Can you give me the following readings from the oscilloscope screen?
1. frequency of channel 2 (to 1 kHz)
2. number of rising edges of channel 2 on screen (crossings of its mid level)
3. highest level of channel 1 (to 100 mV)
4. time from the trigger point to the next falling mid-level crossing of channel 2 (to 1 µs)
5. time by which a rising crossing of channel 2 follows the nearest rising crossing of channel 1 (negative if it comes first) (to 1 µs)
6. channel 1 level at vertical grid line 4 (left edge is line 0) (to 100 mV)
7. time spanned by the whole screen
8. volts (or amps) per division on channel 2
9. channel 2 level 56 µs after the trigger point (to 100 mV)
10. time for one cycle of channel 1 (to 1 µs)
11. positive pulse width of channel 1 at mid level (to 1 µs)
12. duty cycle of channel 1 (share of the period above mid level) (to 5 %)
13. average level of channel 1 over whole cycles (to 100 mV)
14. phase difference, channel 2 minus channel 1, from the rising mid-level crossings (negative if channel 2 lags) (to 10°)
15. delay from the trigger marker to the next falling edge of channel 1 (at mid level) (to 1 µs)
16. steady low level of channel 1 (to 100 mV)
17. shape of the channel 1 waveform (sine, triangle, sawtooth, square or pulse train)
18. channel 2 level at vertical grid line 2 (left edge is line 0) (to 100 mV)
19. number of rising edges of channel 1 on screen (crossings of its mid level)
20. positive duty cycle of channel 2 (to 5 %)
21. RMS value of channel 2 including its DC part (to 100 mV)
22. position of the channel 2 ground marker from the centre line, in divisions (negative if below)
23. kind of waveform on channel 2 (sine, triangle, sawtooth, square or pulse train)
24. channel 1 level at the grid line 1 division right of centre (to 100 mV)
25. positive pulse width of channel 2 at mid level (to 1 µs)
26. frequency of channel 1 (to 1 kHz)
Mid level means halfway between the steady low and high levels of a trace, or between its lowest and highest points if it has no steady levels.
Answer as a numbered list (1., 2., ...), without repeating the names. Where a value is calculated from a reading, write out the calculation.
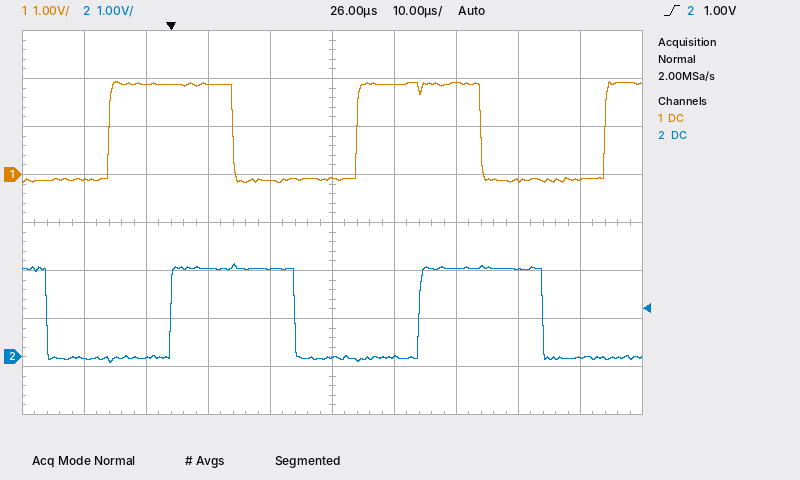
1. 1 / 40 µs ≈ 25 kHz
2. 2
3. 1.9 V
4. 20 µs
5. +10 µs
6. -100 mV
7. 100 µs
8. 1 V
9. 1.8 V
10. 40 µs
11. 20 µs
12. 20 µs / 40 µs ≈ 50 %
13. -100 mV + 0.5 × (1.9 V − (-100 mV)) ≈ 900 mV
14. −360° × (+10 µs) / 40 µs ≈ -90°
15. 10 µs
16. -100 mV
17. square
18. 0.0 V
19. 3
20. 20 µs / 40 µs ≈ 50 %
21. √(0.5 × (1.9 V)² + 0.5 × (-100 mV)²) ≈ 1.3 V
22. -2.8 div
23. square
24. 1.9 V
25. 20 µs
26. 1 / 40 µs ≈ 25 kHz
